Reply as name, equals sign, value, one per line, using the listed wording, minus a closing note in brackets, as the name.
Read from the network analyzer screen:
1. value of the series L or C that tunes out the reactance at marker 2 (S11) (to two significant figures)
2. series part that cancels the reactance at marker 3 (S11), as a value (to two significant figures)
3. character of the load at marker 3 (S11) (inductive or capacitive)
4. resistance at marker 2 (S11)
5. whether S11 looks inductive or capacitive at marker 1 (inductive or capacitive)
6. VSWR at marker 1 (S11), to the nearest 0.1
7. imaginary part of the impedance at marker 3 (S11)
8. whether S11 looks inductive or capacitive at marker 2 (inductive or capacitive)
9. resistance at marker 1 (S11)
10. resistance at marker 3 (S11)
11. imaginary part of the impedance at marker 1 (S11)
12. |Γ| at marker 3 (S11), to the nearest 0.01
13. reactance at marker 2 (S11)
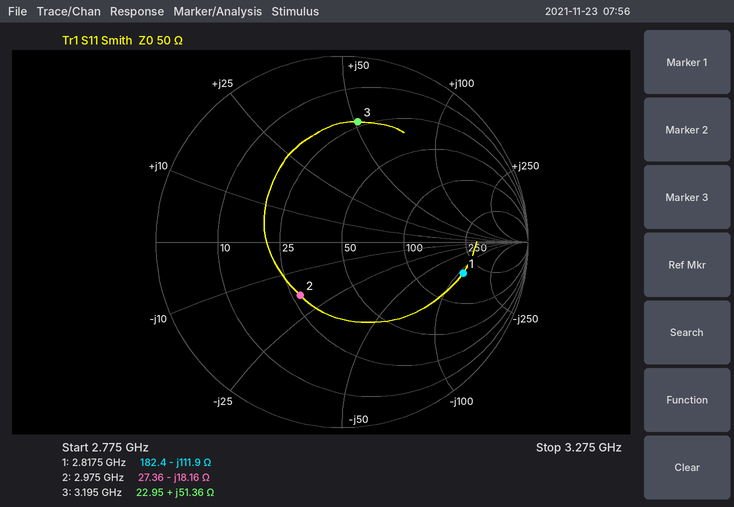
value of the series L or C that tunes out the reactance at marker 2 (S11) = 970 pH
series part that cancels the reactance at marker 3 (S11), as a value = 970 fF
character of the load at marker 3 (S11) = inductive
resistance at marker 2 = 27.36 Ω
whether S11 looks inductive or capacitive at marker 1 = capacitive
VSWR at marker 1 (S11), to the nearest 0.1 = 5.1
imaginary part of the impedance at marker 3 = +51.36 Ω
whether S11 looks inductive or capacitive at marker 2 = capacitive
resistance at marker 1 = 182.4 Ω
resistance at marker 3 = 22.95 Ω
imaginary part of the impedance at marker 1 = -111.9 Ω
|Γ| at marker 3 (S11), to the nearest 0.01 = 0.65
reactance at marker 2 = -18.16 Ω
